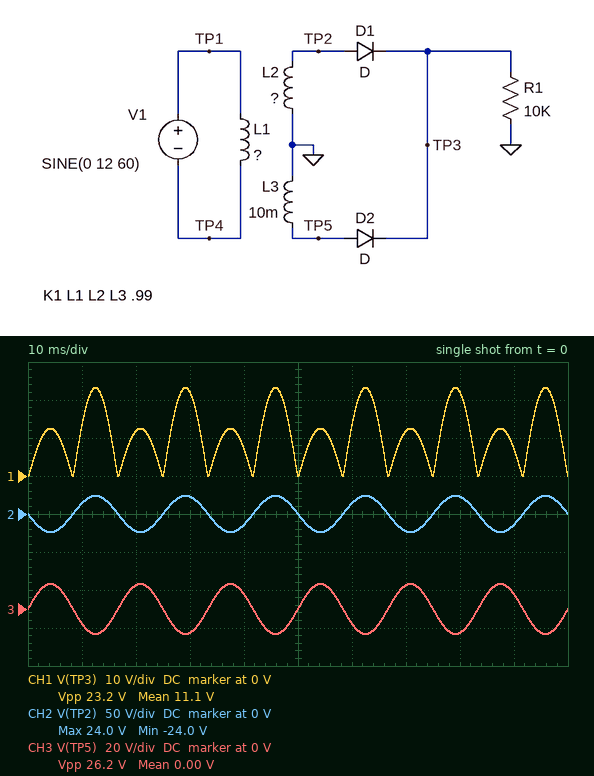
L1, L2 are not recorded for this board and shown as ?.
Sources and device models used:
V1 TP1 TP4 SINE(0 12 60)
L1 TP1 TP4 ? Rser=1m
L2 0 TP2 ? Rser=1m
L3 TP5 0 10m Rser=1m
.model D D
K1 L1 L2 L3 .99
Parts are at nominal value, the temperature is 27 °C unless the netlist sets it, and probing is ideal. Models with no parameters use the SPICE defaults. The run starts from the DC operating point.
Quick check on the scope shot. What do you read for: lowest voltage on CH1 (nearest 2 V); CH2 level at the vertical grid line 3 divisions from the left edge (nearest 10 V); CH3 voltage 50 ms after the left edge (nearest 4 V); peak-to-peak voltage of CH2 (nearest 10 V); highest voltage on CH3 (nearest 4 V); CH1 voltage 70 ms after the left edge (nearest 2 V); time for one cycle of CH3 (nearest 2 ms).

0 V
20 V
0 V
50 V
12 V
12 V
16 ms
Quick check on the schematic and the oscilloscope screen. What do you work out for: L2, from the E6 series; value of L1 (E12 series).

33 mH
8.2 mH
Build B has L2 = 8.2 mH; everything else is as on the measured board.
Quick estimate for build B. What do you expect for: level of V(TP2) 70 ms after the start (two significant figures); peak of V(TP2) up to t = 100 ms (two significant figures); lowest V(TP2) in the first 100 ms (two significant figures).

-11 V
12 V
-12 V
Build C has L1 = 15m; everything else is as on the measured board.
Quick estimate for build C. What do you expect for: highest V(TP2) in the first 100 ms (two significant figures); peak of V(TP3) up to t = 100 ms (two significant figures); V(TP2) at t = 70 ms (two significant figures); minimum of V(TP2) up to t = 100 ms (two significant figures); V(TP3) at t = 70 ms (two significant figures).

18 V
17 V
-17 V
-18 V
8.6 V
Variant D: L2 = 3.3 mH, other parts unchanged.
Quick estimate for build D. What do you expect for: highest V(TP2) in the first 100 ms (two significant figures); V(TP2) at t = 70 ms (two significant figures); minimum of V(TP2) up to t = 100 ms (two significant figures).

7.5 V
-7.2 V
-7.5 V
